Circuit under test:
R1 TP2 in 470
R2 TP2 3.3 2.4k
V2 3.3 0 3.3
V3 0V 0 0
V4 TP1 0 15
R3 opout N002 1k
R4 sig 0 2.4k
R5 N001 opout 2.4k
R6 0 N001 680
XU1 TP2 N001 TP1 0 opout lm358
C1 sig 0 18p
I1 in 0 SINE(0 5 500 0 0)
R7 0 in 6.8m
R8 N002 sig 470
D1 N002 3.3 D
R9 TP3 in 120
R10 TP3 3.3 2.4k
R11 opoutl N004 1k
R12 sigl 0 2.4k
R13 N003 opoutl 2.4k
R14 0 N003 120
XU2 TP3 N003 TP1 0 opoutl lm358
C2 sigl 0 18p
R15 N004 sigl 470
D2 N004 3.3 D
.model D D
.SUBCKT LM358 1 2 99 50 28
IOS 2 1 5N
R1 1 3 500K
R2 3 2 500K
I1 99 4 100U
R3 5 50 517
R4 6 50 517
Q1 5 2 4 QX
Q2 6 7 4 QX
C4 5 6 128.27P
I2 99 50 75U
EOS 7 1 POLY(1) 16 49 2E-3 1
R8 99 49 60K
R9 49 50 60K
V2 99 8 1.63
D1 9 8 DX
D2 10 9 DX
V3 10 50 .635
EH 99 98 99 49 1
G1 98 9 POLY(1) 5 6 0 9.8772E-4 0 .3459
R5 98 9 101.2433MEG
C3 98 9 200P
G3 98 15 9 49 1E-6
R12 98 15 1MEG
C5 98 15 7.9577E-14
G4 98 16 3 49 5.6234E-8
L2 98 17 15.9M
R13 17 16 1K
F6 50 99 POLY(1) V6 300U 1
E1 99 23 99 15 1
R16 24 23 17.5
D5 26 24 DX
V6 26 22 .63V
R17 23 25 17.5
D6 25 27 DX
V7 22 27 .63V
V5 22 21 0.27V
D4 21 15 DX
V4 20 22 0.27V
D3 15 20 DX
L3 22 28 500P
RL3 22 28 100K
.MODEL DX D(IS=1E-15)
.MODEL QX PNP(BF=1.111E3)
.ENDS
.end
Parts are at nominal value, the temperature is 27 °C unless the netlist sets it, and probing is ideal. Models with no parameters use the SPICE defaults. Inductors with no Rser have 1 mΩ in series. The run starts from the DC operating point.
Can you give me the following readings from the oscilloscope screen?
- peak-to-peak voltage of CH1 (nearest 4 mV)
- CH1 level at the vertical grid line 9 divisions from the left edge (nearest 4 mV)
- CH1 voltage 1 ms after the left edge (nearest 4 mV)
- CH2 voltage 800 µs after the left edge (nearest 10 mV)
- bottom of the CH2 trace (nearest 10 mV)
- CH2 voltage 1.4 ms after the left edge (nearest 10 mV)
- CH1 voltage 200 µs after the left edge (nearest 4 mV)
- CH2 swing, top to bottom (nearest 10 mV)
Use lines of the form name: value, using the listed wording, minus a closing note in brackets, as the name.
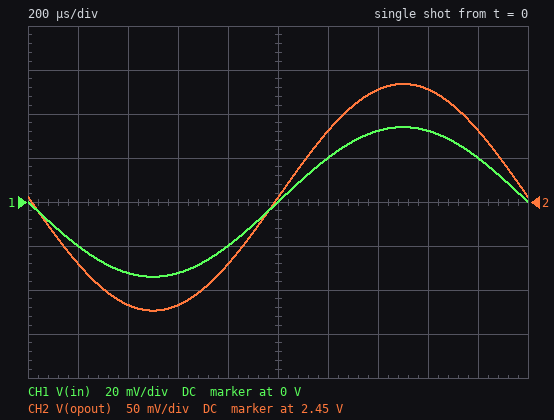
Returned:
peak-to-peak voltage of CH1: 68 mV
CH1 level at the vertical grid line 9 divisions from the left edge: 20 mV
CH1 voltage 1 ms after the left edge: 0 V
CH2 voltage 800 µs after the left edge: 2.38 V
bottom of the CH2 trace: 2.33 V
CH2 voltage 1.4 ms after the left edge: 2.58 V
CH1 voltage 200 µs after the left edge: -20 mV
CH2 swing, top to bottom: 260 mV
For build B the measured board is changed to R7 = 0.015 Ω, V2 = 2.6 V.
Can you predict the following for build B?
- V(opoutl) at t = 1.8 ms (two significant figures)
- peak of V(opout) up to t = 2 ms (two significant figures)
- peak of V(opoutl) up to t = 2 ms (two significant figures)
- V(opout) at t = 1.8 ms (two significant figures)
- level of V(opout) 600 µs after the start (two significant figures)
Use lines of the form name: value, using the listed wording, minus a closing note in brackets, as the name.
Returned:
V(opoutl) at t = 1.8 ms: 3.5 V
peak of V(opout) up to t = 2 ms: 2.2 V
peak of V(opoutl) up to t = 2 ms: 4.1 V
V(opout) at t = 1.8 ms: 2.1 V
level of V(opout) 600 µs after the start: 1.7 V
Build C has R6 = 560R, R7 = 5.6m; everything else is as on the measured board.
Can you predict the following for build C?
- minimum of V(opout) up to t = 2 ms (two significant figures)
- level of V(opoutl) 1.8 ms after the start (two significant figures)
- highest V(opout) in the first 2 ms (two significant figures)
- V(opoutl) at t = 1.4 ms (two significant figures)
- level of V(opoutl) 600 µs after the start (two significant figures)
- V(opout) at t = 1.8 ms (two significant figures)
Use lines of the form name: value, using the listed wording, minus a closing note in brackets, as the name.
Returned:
minimum of V(opout) up to t = 2 ms: 2.7 V
level of V(opoutl) 1.8 ms after the start: 3.7 V
highest V(opout) in the first 2 ms: 3.0 V
V(opoutl) at t = 1.4 ms: 3.9 V
level of V(opoutl) 600 µs after the start: 2.8 V
V(opout) at t = 1.8 ms: 2.9 V
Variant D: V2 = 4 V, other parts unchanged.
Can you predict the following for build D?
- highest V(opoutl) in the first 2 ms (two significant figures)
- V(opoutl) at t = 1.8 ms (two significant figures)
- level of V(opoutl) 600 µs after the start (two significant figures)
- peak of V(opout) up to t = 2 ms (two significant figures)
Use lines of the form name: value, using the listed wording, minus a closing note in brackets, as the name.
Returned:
highest V(opoutl) in the first 2 ms: 4.7 V
V(opoutl) at t = 1.8 ms: 4.4 V
level of V(opoutl) 600 µs after the start: 3.4 V
peak of V(opout) up to t = 2 ms: 3.1 V
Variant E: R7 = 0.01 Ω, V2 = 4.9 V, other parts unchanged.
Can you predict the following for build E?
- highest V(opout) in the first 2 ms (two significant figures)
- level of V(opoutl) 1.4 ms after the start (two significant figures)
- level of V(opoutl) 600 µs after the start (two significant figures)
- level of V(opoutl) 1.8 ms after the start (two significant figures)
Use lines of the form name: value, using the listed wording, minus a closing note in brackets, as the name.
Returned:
highest V(opout) in the first 2 ms: 3.8 V
level of V(opoutl) 1.4 ms after the start: 5.9 V
level of V(opoutl) 600 µs after the start: 4.0 V
level of V(opoutl) 1.8 ms after the start: 5.5 V
